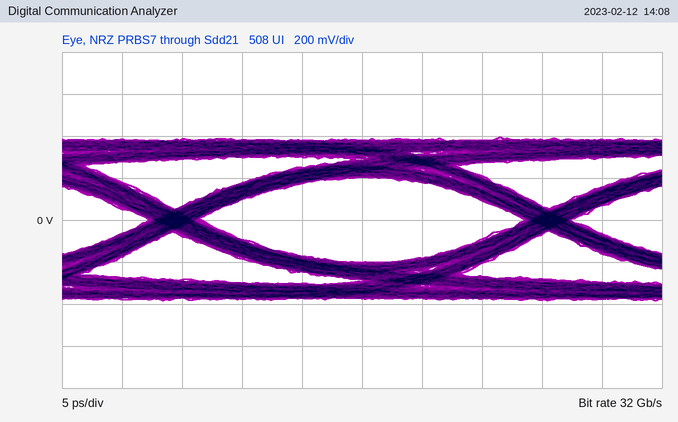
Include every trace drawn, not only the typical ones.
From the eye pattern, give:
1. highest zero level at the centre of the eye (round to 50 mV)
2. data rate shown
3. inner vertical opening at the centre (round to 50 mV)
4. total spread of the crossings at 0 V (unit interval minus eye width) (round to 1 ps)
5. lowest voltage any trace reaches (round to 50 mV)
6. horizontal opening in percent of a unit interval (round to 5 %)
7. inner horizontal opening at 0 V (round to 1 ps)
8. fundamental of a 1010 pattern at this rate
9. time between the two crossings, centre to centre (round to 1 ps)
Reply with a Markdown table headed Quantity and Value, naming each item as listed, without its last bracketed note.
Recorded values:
| Quantity | Value |
|---|---|
| highest zero level at the centre of the eye | -200 mV |
| data rate shown | 32 Gb/s |
| inner vertical opening at the centre | 400 mV |
| total spread of the crossings at 0 V (unit interval minus eye width) | 4 ps |
| lowest voltage any trace reaches | -400 mV |
| horizontal opening in percent of a unit interval | 85 % |
| inner horizontal opening at 0 V | 27 ps |
| fundamental of a 1010 pattern at this rate | 16 GHz |
| time between the two crossings, centre to centre | 31 ps |
